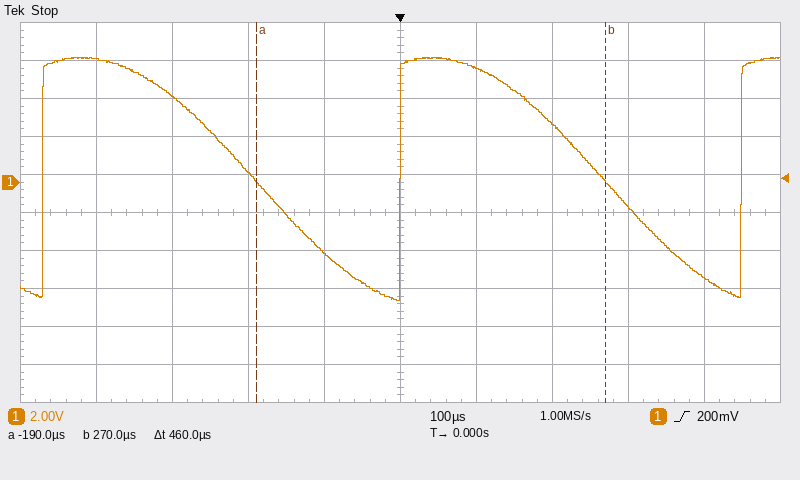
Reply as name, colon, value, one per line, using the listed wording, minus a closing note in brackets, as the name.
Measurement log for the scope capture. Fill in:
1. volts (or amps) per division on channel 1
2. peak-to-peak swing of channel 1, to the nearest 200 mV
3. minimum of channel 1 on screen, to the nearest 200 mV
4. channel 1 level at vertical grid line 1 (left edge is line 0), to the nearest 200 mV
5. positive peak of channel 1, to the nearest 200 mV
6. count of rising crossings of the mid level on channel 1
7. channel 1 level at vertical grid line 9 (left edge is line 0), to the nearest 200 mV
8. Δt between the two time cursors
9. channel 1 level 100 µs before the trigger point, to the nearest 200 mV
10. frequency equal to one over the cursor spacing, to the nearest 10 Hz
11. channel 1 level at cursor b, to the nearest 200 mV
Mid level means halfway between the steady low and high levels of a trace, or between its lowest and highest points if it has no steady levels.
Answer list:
volts (or amps) per division on channel 1: 2 V
peak-to-peak swing of channel 1, to the nearest 200 mV: 12.8 V
minimum of channel 1 on screen, to the nearest 200 mV: -6.2 V
channel 1 level at vertical grid line 1 (left edge is line 0), to the nearest 200 mV: 6.4 V
positive peak of channel 1, to the nearest 200 mV: 6.6 V
count of rising crossings of the mid level on channel 1: 3
channel 1 level at vertical grid line 9 (left edge is line 0), to the nearest 200 mV: -5.0 V
Δt between the two time cursors: 460 µs
channel 1 level 100 µs before the trigger point, to the nearest 200 mV: -3.8 V
frequency equal to one over the cursor spacing, to the nearest 10 Hz: 2.17 kHz
channel 1 level at cursor b, to the nearest 200 mV: 0.0 V
